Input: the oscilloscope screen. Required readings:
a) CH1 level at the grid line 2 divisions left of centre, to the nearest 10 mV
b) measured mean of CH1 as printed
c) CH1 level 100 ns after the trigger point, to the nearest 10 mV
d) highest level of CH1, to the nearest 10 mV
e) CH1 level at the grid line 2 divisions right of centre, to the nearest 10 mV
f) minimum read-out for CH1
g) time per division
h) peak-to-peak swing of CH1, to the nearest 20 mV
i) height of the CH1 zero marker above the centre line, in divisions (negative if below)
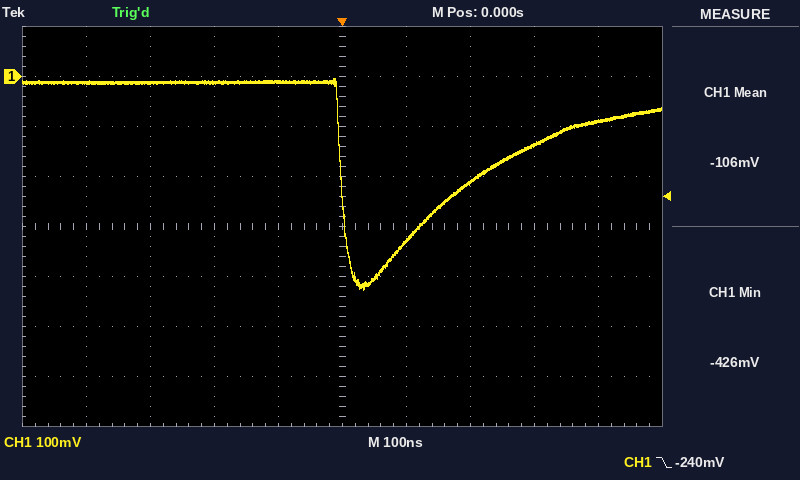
-10 mV
-106 mV
-330 mV
0 mV
-210 mV
-426 mV
100 ns
420 mV
+3.0 div
